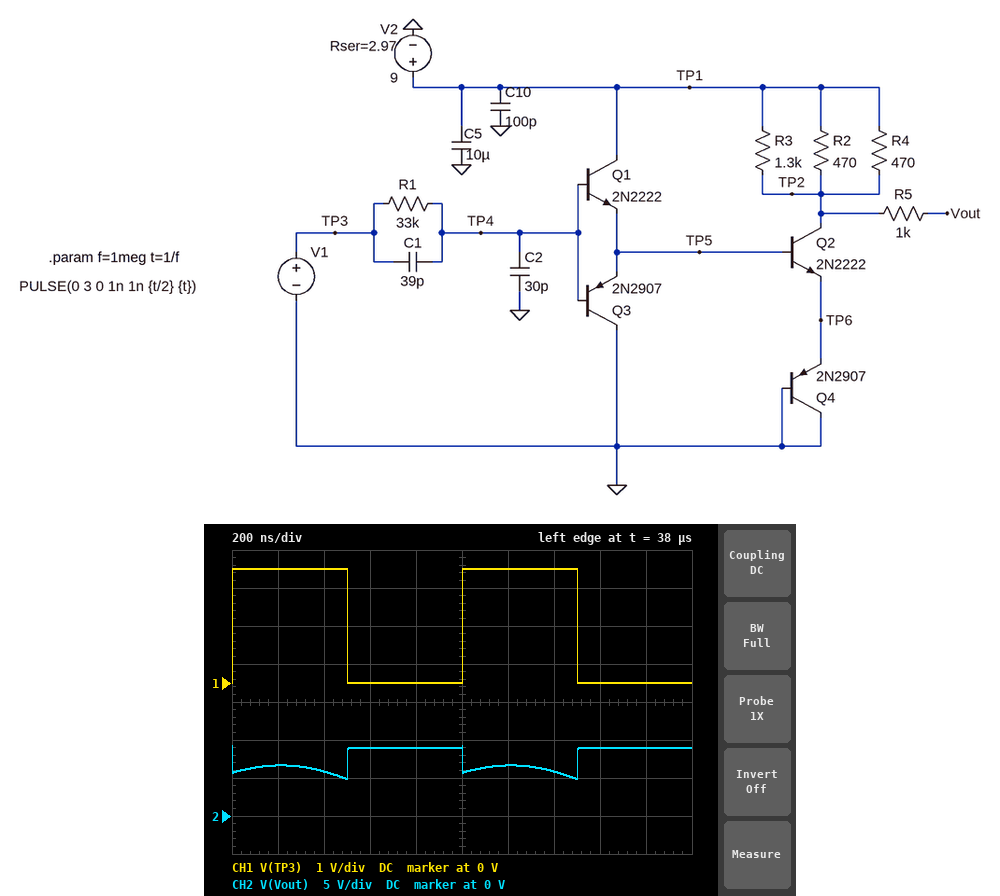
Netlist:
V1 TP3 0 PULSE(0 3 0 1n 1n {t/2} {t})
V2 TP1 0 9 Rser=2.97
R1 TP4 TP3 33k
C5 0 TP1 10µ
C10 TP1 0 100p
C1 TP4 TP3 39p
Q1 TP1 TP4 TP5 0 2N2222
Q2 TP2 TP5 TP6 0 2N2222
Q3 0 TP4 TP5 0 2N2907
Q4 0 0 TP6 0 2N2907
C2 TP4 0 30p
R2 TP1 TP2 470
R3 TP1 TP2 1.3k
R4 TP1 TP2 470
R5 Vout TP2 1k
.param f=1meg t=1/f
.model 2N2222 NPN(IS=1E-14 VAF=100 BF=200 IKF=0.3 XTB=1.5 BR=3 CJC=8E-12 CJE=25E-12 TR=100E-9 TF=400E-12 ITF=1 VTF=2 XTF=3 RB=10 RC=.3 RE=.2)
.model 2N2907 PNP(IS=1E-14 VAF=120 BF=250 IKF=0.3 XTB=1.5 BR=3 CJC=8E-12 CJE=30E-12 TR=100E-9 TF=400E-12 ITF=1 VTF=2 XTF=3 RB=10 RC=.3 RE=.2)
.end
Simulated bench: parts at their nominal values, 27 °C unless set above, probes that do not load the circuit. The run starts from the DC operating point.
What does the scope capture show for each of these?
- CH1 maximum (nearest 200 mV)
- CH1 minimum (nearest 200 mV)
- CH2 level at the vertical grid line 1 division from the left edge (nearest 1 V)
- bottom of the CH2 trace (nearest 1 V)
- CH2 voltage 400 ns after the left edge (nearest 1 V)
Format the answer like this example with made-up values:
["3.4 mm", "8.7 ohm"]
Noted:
["3.0 V", "0 V", "7 V", "5 V", "6 V"]
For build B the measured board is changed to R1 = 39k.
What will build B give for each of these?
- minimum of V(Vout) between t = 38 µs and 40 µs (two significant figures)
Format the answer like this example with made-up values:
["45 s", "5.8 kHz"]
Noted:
["5.0 V"]
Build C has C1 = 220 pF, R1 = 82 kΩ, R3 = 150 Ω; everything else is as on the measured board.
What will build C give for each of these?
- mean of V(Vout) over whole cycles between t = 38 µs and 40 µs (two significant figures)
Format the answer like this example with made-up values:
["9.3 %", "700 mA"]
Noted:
["4.9 V"]
